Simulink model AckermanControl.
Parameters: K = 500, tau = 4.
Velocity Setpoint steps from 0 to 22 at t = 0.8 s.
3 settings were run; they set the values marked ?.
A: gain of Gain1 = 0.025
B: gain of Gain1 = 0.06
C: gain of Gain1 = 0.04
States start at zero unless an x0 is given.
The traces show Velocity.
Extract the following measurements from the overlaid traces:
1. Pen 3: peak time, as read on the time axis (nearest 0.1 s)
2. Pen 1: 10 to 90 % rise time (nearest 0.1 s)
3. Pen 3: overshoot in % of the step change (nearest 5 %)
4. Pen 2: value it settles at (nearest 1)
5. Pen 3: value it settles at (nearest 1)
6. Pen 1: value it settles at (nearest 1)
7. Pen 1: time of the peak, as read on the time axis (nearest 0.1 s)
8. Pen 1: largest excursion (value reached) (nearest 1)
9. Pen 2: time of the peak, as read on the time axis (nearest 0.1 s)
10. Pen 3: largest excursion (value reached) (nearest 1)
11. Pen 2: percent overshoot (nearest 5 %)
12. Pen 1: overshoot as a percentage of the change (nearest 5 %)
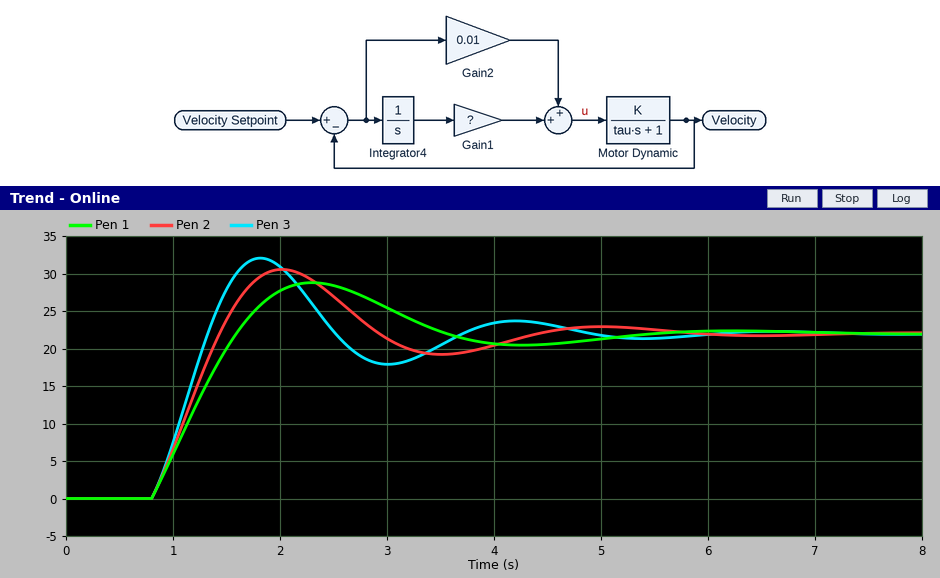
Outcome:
1.8 s
0.6 s
45 %
22
22
22
2.3 s
29
2.0 s
32
40 %
30 %
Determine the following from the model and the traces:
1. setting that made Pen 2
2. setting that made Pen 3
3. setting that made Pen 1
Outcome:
C
B
A
